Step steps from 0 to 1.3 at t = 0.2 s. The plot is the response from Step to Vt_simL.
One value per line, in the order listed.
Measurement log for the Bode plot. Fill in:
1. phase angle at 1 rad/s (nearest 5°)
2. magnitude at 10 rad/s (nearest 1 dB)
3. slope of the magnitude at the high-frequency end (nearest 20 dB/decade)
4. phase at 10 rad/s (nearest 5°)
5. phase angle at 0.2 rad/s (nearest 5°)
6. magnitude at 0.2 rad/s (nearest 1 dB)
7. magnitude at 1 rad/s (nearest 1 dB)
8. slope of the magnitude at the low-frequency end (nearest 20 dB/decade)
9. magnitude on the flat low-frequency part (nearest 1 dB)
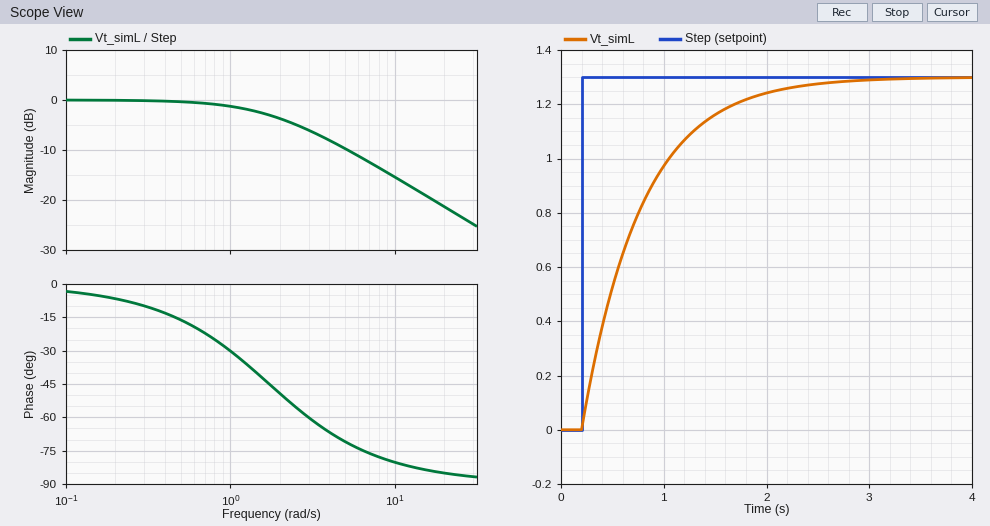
-30°
-15 dB
-20 dB/decade
-80°
-5°
0 dB
-1 dB
0 dB/decade
0 dB
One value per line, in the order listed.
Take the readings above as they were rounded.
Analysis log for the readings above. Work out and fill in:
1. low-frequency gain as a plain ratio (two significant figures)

1.0
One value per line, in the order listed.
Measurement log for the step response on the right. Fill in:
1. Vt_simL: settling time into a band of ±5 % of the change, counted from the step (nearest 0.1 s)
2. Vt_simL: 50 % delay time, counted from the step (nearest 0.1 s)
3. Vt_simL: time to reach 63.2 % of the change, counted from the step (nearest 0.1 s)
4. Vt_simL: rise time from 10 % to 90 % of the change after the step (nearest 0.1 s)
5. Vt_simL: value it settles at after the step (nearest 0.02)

1.7 s
0.4 s
0.6 s
1.3 s
1.30
